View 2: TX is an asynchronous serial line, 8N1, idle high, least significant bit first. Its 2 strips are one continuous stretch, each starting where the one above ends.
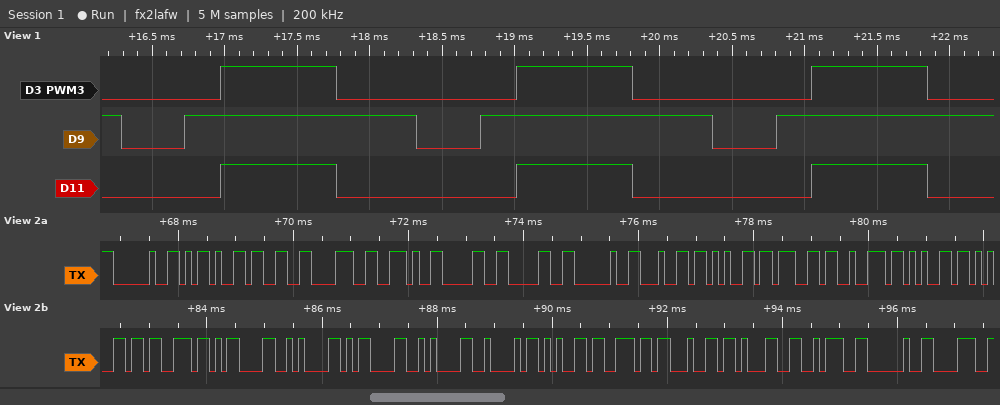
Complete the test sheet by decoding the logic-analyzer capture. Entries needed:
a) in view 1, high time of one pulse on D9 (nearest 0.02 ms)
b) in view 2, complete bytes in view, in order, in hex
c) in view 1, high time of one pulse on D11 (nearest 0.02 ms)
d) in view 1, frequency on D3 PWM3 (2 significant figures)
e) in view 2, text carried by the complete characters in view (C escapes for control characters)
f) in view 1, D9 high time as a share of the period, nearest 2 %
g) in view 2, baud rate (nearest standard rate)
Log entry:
1.60 ms
20 2D 33 38 2E 30 30 20 64 65 67 72 65 65 73 0D 0A 0D 0A 42 65 6E 64 31 3A 20 38
0.80 ms
490 Hz
" -38.00 degrees\r\n\r\nBend1: 8"
78 %
9600 baud
